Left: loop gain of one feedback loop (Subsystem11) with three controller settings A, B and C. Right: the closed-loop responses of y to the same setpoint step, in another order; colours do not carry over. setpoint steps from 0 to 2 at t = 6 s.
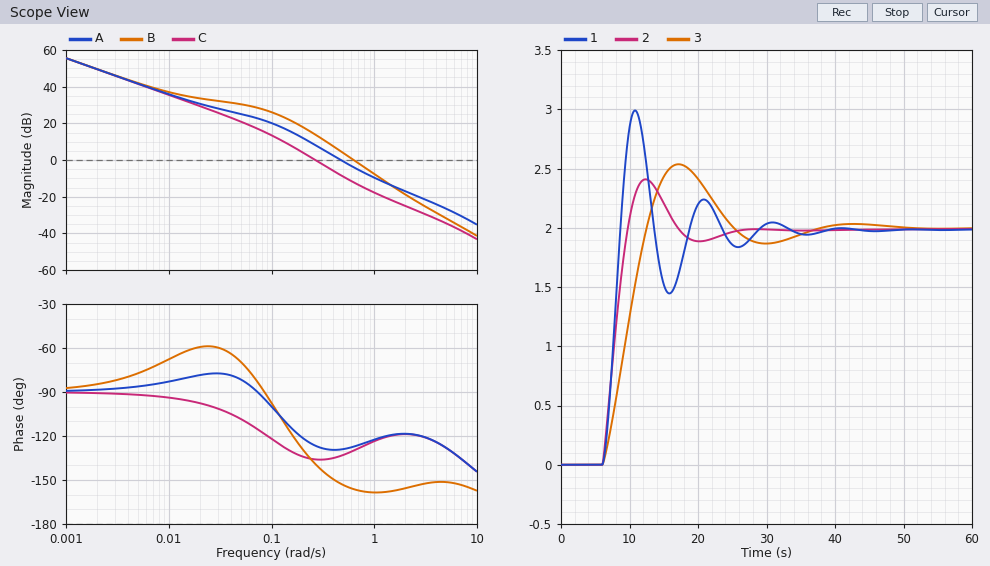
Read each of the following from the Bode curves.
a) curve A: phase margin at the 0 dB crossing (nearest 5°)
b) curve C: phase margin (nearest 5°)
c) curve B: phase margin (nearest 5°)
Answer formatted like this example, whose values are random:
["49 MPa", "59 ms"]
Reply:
["50°", "45°", "25°"]
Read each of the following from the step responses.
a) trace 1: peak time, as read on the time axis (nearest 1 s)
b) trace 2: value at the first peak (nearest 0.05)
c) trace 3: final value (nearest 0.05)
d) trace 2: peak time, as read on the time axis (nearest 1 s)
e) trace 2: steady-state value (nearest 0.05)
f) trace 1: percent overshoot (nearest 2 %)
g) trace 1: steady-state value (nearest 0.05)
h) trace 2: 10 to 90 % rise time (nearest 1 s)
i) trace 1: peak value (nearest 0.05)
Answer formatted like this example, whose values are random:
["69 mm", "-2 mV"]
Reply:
["11 s", "2.40", "2.00", "12 s", "2.00", "50 %", "2.00", "3 s", "3.00"]
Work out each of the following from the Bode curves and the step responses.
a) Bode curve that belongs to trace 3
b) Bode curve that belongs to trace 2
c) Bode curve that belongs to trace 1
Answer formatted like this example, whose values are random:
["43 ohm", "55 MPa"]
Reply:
["C", "A", "B"]
